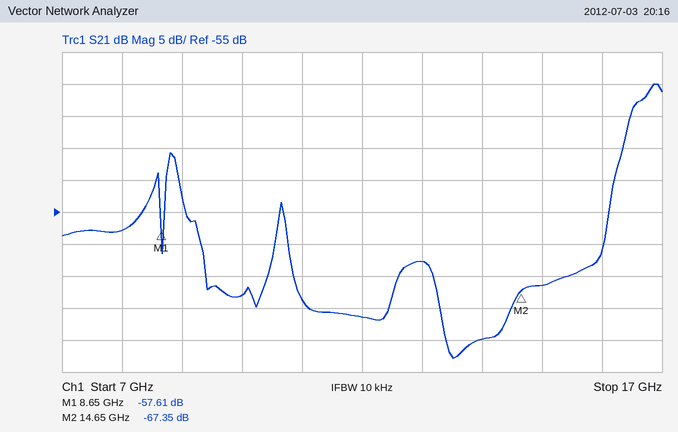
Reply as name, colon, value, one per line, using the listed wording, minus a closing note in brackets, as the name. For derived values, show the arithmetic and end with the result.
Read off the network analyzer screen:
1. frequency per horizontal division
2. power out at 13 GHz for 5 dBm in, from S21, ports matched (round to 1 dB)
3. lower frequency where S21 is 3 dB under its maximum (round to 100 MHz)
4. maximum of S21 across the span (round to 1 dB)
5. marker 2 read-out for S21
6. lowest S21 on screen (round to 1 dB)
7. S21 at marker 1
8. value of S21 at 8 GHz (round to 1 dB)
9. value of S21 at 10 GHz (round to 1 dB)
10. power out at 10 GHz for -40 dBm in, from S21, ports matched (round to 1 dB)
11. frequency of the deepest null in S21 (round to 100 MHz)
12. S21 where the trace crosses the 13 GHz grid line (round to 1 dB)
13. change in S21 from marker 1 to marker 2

frequency per horizontal division: 1 GHz
power out at 13 GHz for 5 dBm in, from S21, ports matched: 5 dBm + (-63 dB) = -58 dBm
lower frequency where S21 is 3 dB under its maximum: 16.6 GHz
maximum of S21 across the span: -35 dB
marker 2 read-out for S21: -67.35 dB
lowest S21 on screen: -78 dB
S21 at marker 1: -57.61 dB
value of S21 at 8 GHz: -58 dB
value of S21 at 10 GHz: -68 dB
power out at 10 GHz for -40 dBm in, from S21, ports matched: -40 dBm + (-68 dB) = -108 dBm
frequency of the deepest null in S21: 13.5 GHz
S21 where the trace crosses the 13 GHz grid line: -63 dB
change in S21 from marker 1 to marker 2: -67.35 − (-57.61) = -9.74 dB
